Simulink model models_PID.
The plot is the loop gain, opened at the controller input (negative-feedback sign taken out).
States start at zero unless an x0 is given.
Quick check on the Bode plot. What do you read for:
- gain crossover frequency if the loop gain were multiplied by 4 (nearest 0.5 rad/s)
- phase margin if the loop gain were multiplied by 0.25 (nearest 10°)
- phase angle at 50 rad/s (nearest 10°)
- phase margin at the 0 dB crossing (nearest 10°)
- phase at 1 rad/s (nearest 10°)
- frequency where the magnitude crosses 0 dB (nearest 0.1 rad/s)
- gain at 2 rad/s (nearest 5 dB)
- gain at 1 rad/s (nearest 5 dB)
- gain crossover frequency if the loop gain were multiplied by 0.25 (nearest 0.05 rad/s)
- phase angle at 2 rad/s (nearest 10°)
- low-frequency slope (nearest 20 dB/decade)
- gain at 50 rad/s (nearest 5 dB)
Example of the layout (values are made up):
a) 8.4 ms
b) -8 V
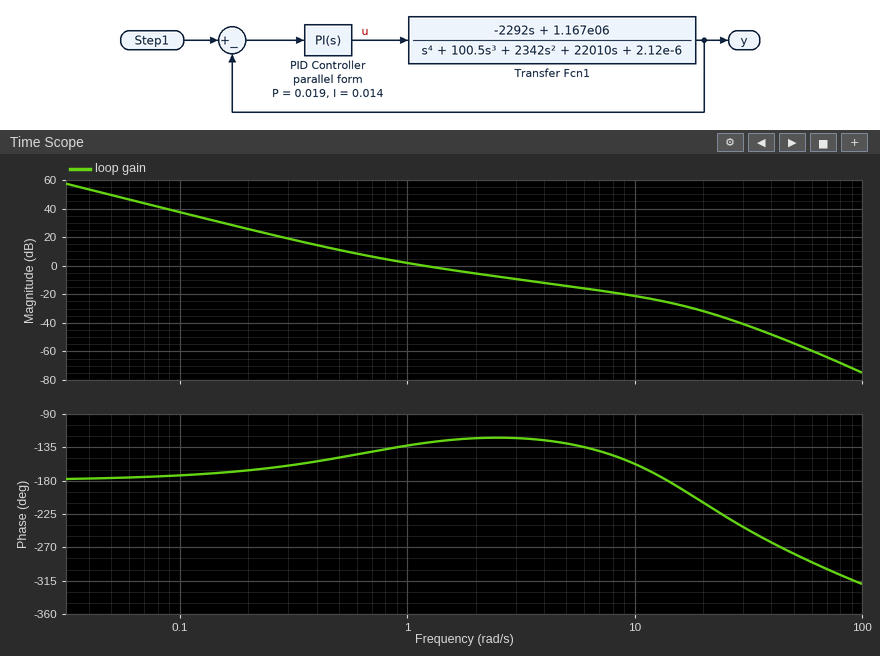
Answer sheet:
a) 4.0 rad/s
b) 30°
c) -280°
d) 50°
e) -130°
f) 1.2 rad/s
g) -5 dB
h) 0 dB
i) 0.45 rad/s
j) -120°
k) -40 dB/decade
l) -55 dB
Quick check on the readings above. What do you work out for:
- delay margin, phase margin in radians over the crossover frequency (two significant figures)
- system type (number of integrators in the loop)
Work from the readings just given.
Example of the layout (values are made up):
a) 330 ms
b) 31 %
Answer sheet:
a) 0.73 s
b) 2
